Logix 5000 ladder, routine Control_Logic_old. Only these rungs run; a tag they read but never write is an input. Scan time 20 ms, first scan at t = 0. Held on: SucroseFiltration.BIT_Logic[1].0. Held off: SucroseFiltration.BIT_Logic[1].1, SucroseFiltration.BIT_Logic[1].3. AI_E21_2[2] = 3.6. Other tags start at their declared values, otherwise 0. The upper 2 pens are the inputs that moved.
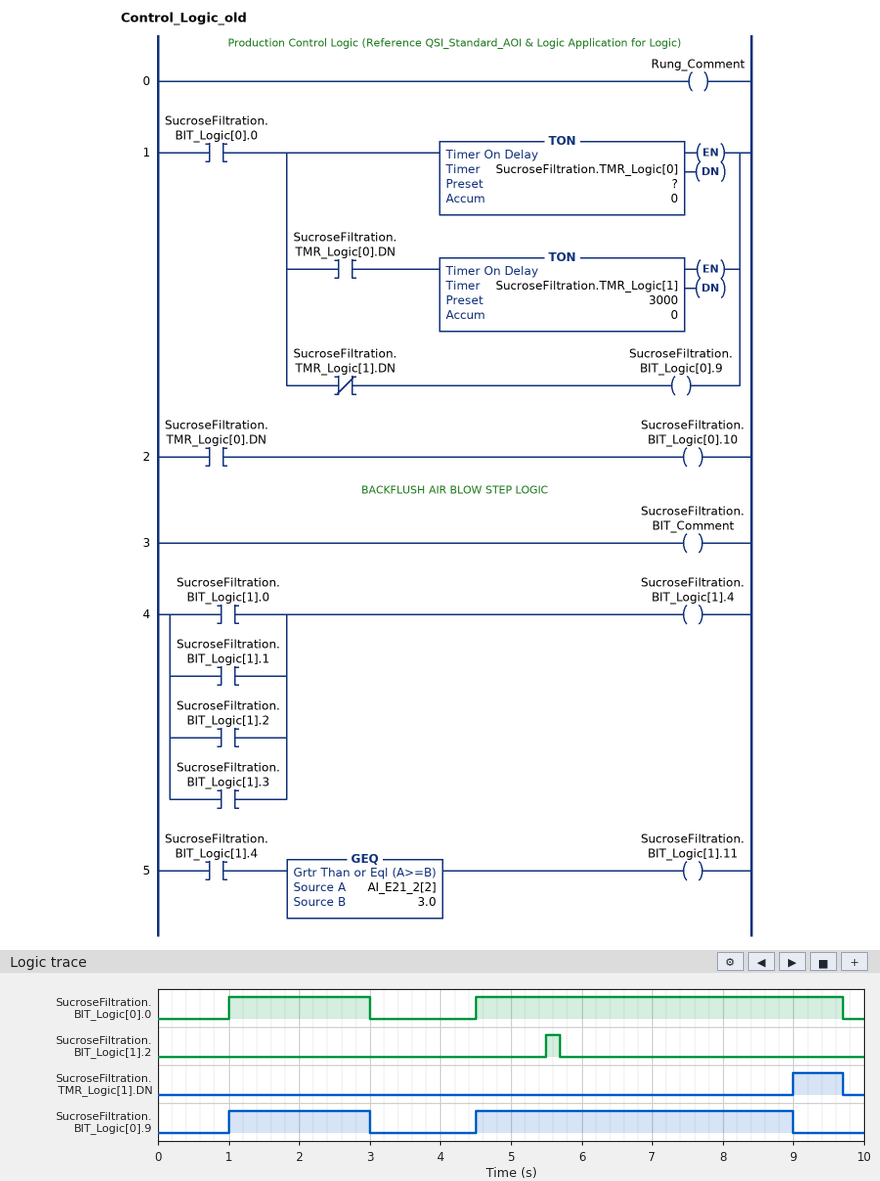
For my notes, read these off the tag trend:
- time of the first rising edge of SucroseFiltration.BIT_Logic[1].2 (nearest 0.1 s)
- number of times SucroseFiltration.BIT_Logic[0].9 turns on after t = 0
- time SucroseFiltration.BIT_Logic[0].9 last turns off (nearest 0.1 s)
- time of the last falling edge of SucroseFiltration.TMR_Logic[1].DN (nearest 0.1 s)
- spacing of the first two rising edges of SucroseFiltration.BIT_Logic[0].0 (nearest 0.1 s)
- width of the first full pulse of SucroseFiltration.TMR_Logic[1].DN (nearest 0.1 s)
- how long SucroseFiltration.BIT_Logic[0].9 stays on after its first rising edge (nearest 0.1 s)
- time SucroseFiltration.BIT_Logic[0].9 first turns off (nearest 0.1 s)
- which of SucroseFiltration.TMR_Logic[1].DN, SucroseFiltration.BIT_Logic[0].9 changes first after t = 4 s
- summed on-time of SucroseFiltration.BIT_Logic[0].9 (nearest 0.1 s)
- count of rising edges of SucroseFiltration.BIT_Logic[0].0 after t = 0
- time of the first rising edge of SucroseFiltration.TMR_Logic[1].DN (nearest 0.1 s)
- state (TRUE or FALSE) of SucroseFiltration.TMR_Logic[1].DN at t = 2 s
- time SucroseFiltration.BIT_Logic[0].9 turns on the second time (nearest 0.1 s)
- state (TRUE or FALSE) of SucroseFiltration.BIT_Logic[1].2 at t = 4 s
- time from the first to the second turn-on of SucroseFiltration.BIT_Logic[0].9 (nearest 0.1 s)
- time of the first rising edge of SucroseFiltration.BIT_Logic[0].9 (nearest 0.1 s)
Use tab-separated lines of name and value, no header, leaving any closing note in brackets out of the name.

time of the first rising edge of SucroseFiltration.BIT_Logic[1].2	5.5 s
number of times SucroseFiltration.BIT_Logic[0].9 turns on after t = 0	2
time SucroseFiltration.BIT_Logic[0].9 last turns off	9.0 s
time of the last falling edge of SucroseFiltration.TMR_Logic[1].DN	9.7 s
spacing of the first two rising edges of SucroseFiltration.BIT_Logic[0].0	3.5 s
width of the first full pulse of SucroseFiltration.TMR_Logic[1].DN	0.7 s
how long SucroseFiltration.BIT_Logic[0].9 stays on after its first rising edge	2.0 s
time SucroseFiltration.BIT_Logic[0].9 first turns off	3.0 s
which of SucroseFiltration.TMR_Logic[1].DN, SucroseFiltration.BIT_Logic[0].9 changes first after t = 4 s	SucroseFiltration.BIT_Logic[0].9
summed on-time of SucroseFiltration.BIT_Logic[0].9	6.5 s
count of rising edges of SucroseFiltration.BIT_Logic[0].0 after t = 0	2
time of the first rising edge of SucroseFiltration.TMR_Logic[1].DN	9.0 s
state (TRUE or FALSE) of SucroseFiltration.TMR_Logic[1].DN at t = 2 s	FALSE
time SucroseFiltration.BIT_Logic[0].9 turns on the second time	4.5 s
state (TRUE or FALSE) of SucroseFiltration.BIT_Logic[1].2 at t = 4 s	FALSE
time from the first to the second turn-on of SucroseFiltration.BIT_Logic[0].9	3.5 s
time of the first rising edge of SucroseFiltration.BIT_Logic[0].9	1.0 s
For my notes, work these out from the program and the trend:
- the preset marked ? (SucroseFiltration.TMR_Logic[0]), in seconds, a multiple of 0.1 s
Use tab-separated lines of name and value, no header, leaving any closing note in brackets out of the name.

the preset marked ? (SucroseFiltration.TMR_Logic[0]), in seconds, a multiple of 0.1 s	1.5 s
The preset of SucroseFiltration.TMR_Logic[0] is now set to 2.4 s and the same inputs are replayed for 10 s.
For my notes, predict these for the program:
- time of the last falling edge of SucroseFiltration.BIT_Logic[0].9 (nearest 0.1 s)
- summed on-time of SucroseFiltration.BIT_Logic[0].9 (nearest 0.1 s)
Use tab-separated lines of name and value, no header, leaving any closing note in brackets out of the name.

time of the last falling edge of SucroseFiltration.BIT_Logic[0].9	9.7 s
summed on-time of SucroseFiltration.BIT_Logic[0].9	7.2 s
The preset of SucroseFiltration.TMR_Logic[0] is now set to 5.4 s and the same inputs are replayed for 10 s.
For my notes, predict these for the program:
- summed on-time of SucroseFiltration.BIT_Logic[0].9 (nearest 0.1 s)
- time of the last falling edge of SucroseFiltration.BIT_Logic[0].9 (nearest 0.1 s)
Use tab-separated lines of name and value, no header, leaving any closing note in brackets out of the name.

summed on-time of SucroseFiltration.BIT_Logic[0].9	7.2 s
time of the last falling edge of SucroseFiltration.BIT_Logic[0].9	9.7 s
